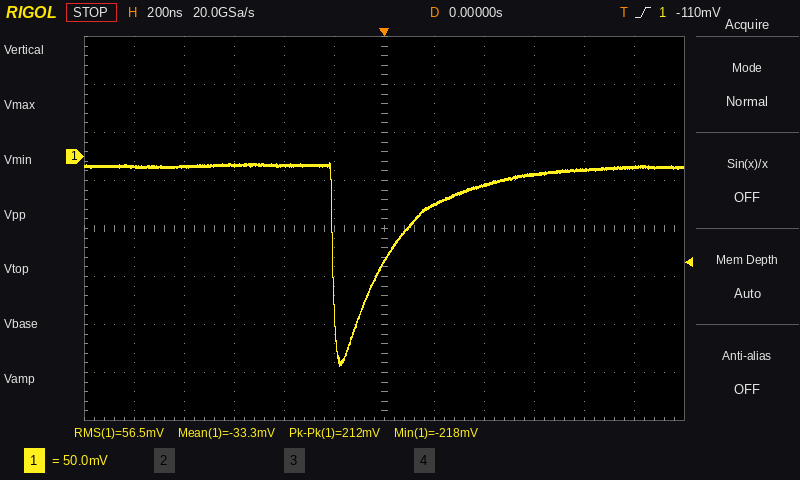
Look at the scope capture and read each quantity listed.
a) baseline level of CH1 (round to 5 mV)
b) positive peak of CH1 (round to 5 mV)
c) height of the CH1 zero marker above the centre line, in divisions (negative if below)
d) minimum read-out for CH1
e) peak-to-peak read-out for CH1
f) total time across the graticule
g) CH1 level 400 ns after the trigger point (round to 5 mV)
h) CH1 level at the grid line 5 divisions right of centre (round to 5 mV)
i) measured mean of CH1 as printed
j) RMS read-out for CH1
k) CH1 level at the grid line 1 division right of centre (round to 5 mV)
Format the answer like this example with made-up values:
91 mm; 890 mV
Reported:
-10 mV; -5 mV; +1.5 div; -218 mV; 212 mV; 2.4 µs; -30 mV; -10 mV; -33.3 mV; 56.5 mV; -50 mV
